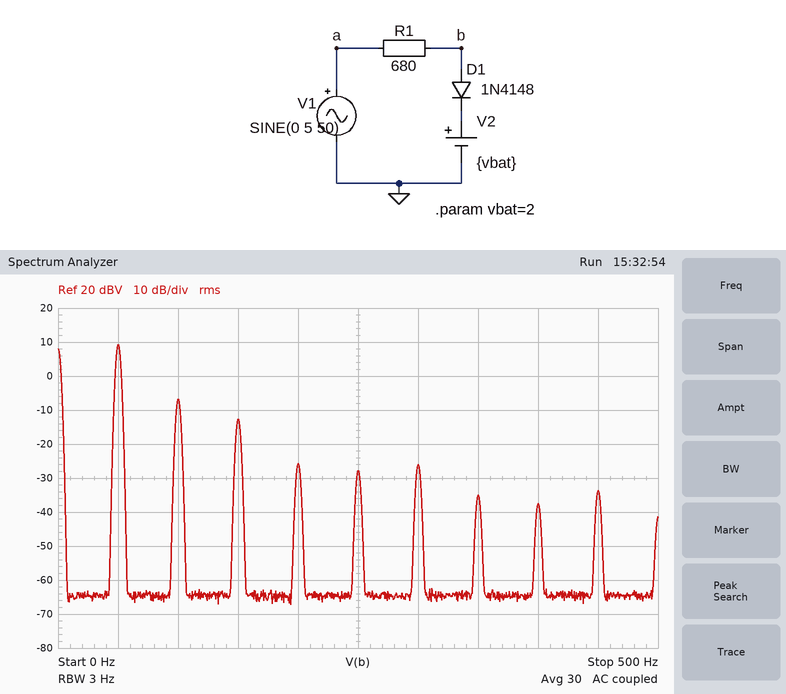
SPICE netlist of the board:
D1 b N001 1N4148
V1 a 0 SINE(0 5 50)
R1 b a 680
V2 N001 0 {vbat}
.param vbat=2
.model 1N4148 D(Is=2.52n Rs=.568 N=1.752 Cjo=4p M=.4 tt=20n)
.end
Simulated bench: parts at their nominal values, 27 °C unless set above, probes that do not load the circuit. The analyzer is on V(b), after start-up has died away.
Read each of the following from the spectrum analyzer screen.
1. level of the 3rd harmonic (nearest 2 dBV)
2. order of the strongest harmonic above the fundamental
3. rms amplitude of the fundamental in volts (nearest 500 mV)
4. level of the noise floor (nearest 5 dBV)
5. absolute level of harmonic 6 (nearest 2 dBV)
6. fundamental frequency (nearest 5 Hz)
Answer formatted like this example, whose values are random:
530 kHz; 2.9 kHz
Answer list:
-12 dBV; 2; 3.0 V; -65 dBV; -26 dBV; 50 Hz
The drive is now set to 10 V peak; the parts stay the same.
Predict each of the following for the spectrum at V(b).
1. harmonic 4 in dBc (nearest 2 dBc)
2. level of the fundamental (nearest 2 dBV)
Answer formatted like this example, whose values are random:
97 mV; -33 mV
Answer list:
-30 dBc; 14 dBV
